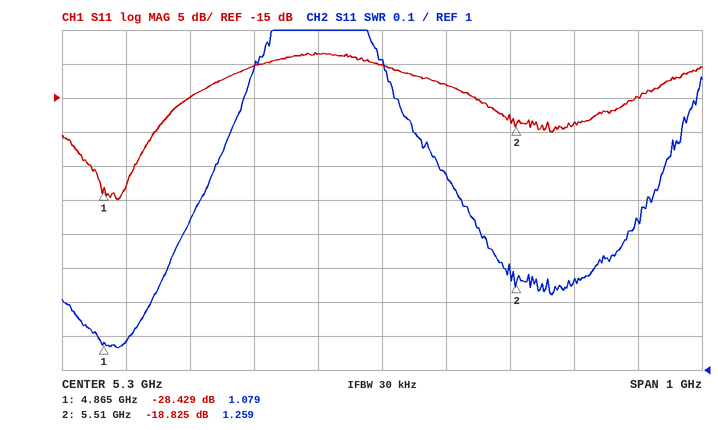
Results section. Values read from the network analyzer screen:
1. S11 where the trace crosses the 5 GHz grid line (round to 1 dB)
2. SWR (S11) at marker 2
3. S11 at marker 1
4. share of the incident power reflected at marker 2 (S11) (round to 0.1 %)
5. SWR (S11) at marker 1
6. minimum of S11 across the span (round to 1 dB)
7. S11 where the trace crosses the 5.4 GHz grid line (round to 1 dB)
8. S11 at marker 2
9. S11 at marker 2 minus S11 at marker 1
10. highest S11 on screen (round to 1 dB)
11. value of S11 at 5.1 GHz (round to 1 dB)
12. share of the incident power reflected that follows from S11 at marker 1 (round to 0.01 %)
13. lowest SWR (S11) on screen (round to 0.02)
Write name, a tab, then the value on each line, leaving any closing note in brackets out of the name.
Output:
S11 where the trace crosses the 5 GHz grid line	-15 dB
SWR (S11) at marker 2	1.259
S11 at marker 1	-28.429 dB
share of the incident power reflected at marker 2 (S11)	1.3 %
SWR (S11) at marker 1	1.079
minimum of S11 across the span	-30 dB
S11 where the trace crosses the 5.4 GHz grid line	-13 dB
S11 at marker 2	-18.825 dB
S11 at marker 2 minus S11 at marker 1	9.604 dB
highest S11 on screen	-8 dB
value of S11 at 5.1 GHz	-10 dB
share of the incident power reflected that follows from S11 at marker 1	0.14 %
lowest SWR (S11) on screen	1.06
